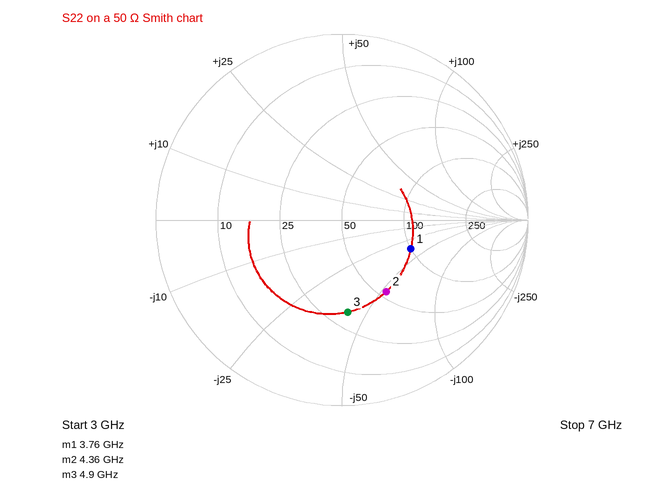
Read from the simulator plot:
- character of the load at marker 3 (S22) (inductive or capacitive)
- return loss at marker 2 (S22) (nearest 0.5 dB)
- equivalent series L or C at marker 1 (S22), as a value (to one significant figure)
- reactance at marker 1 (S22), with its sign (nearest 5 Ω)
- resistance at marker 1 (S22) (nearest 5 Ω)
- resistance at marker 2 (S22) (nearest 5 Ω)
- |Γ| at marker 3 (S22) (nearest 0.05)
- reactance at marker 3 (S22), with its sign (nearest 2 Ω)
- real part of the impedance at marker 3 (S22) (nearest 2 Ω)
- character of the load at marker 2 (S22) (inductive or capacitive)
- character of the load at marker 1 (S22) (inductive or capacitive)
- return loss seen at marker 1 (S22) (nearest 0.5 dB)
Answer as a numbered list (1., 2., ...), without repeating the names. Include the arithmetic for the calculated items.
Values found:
1. capacitive
2. 7.0 dB
3. C = 1/(2π × 3.76 GHz × 35 Ω) ≈ 1 pF
4. -35 Ω
5. 100 Ω
6. 55 Ω
7. 0.50
8. -42 Ω
9. 32 Ω
10. capacitive
11. capacitive
12. 8.0 dB
